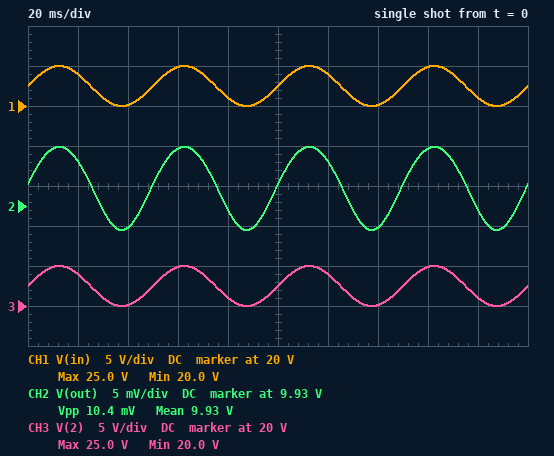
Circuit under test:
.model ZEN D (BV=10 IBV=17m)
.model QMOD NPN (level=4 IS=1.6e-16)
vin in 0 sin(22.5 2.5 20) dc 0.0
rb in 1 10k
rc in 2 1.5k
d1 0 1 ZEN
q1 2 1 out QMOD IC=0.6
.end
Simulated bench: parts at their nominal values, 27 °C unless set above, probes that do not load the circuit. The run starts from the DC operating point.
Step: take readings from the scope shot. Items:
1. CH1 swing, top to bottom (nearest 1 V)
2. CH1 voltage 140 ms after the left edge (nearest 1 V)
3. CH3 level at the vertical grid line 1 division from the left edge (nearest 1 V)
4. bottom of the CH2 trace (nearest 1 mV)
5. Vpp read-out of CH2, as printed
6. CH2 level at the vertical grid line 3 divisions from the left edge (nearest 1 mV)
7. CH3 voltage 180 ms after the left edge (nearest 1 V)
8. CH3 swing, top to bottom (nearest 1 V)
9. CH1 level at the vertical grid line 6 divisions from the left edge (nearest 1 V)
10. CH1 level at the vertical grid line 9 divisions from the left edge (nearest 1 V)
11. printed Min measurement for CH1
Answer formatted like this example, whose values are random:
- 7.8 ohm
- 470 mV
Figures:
- 5 V
- 20 V
- 24 V
- 9.927 V
- 10.4 mV
- 9.937 V
- 21 V
- 5 V
- 24 V
- 21 V
- 20.0 V
